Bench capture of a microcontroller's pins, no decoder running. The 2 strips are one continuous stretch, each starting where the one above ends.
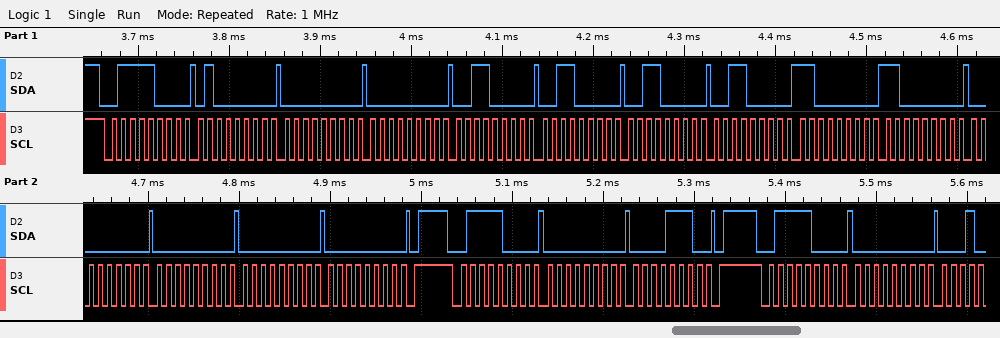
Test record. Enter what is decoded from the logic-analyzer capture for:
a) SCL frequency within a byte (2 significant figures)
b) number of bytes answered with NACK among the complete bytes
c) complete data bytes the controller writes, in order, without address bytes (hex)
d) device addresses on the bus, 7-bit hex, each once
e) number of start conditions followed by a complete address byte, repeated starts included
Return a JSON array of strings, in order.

["100 kHz", "0", "40 00 00 30 30 30 30 C0 C0 00 00 00 00 00 0E 00", "0x3C", "3"]
